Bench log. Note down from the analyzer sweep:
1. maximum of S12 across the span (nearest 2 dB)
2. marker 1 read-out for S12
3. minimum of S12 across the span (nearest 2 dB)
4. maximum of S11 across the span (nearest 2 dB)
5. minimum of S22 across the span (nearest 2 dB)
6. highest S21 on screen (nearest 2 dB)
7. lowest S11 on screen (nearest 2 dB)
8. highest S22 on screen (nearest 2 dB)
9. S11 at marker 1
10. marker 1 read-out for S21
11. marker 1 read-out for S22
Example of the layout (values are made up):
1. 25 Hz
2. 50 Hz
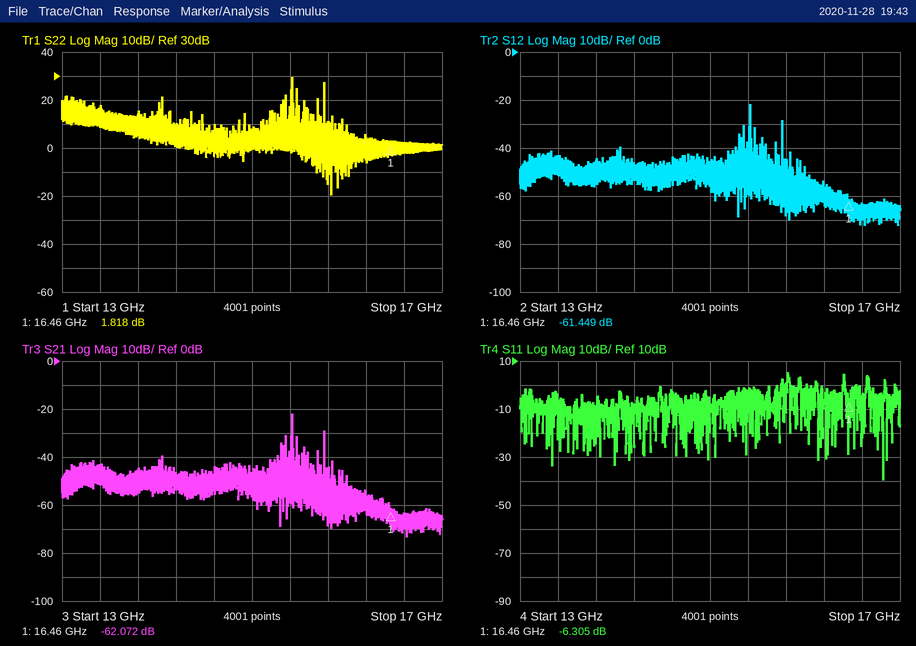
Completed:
1. -22 dB
2. -61.449 dB
3. -72 dB
4. 6 dB
5. -20 dB
6. -22 dB
7. -40 dB
8. 30 dB
9. -6.305 dB
10. -62.072 dB
11. 1.818 dB
